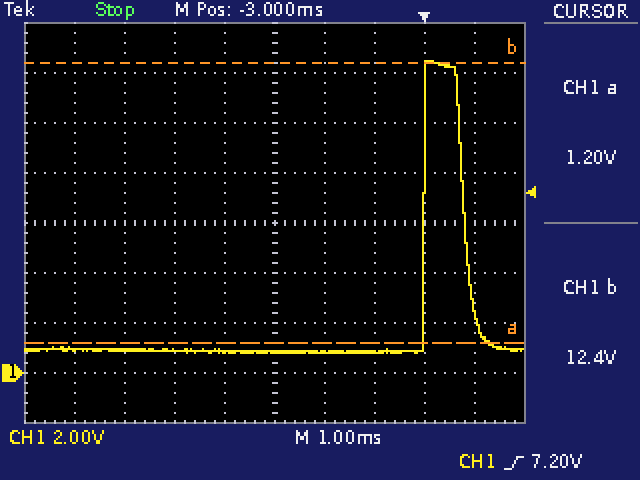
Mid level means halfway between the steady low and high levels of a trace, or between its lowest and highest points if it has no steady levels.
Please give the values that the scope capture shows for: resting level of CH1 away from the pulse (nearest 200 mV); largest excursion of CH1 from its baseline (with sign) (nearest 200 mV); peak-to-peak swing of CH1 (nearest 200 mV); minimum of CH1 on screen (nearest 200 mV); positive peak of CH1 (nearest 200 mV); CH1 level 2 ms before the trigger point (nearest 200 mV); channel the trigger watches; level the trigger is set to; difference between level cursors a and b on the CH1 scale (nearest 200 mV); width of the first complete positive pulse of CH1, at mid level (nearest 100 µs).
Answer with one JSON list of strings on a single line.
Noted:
["800 mV", "+11.6 V", "11.6 V", "800 mV", "12.4 V", "800 mV", "CH1", "7.20 V", "11.2 V", "800 µs"]
